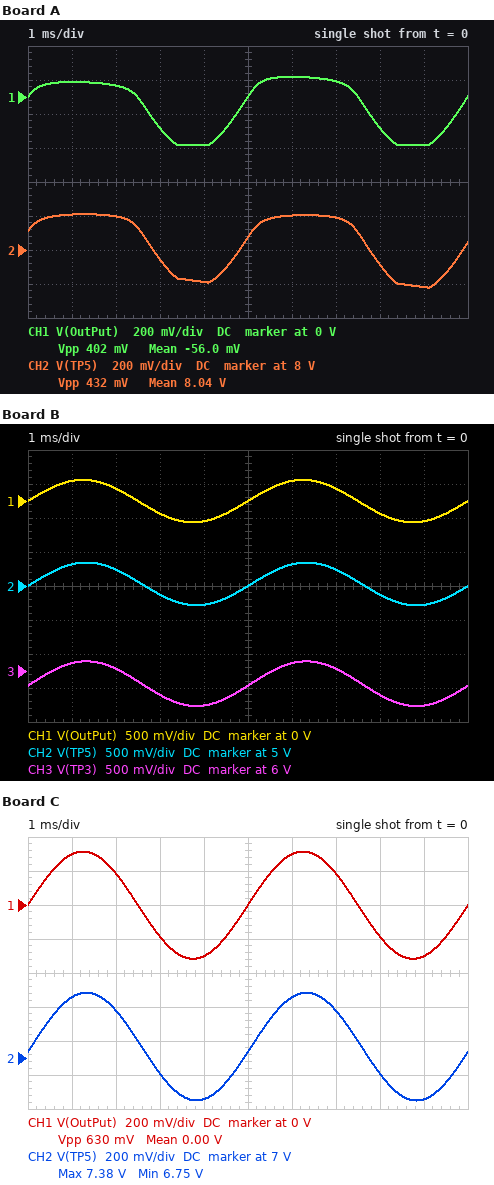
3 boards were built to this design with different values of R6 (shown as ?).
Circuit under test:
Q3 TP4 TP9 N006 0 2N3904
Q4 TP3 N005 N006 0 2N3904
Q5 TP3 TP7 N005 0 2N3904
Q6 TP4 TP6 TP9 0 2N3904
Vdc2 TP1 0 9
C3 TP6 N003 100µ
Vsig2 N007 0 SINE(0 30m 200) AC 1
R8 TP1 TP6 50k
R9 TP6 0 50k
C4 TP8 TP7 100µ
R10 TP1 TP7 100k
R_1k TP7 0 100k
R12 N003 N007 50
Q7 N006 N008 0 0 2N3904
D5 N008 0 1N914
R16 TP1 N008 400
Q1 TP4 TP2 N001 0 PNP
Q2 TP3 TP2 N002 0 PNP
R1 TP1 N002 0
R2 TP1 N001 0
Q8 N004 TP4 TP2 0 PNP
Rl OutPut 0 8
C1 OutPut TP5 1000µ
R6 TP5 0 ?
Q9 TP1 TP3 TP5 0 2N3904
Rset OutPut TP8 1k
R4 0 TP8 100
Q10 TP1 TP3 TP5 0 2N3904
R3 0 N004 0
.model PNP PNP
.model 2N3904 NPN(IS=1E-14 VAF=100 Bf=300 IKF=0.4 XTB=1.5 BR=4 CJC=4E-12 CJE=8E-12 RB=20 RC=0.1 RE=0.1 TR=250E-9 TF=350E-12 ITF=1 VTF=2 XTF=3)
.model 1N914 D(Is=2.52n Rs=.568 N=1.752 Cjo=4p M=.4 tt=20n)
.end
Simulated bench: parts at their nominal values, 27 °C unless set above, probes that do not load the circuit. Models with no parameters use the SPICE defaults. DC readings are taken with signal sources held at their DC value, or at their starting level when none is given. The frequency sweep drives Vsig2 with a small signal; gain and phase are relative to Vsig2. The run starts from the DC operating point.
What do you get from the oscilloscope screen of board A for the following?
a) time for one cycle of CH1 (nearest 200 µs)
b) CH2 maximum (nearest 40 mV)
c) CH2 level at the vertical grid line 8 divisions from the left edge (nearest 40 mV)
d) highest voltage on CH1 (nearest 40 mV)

5.0 ms
8.20 V
7.92 V
120 mV
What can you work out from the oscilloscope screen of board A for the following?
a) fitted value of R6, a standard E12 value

220 Ω
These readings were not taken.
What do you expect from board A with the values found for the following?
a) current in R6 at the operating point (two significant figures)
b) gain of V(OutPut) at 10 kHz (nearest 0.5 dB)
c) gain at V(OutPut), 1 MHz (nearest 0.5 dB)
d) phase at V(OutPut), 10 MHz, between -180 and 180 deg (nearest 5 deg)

37 mA
19.5 dB
19.0 dB
-60 deg
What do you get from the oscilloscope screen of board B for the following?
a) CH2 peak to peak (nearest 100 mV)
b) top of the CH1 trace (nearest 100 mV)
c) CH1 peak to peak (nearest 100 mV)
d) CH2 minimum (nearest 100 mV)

600 mV
300 mV
600 mV
4.7 V
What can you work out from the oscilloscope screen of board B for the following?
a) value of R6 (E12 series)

33 Ω
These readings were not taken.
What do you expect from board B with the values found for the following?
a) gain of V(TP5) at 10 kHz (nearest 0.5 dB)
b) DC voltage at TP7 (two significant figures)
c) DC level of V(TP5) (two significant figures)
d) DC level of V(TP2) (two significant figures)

20.5 dB
4.5 V
5.0 V
8.2 V
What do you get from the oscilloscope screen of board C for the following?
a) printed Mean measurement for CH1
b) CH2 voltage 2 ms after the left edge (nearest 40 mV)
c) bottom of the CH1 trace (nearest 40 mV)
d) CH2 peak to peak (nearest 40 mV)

0.00 V
7.28 V
-320 mV
640 mV
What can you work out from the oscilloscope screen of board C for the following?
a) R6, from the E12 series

82 Ω
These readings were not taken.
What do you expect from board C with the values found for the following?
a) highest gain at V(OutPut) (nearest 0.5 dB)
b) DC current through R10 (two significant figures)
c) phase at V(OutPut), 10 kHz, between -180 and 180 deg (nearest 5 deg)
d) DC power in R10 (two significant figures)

20.5 dB
45 µA
0 deg
200 µW
